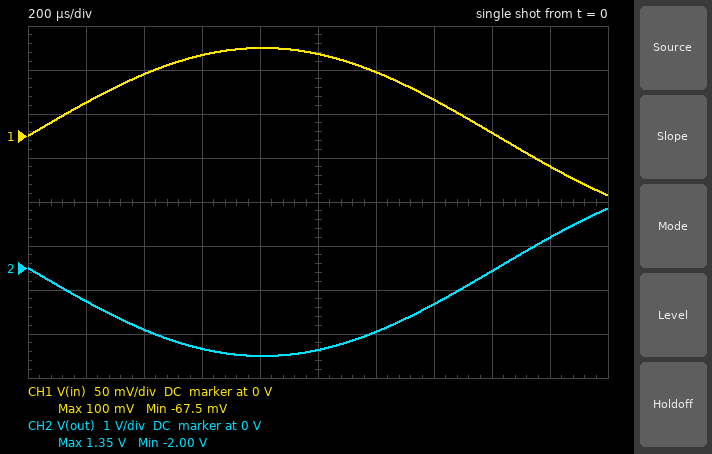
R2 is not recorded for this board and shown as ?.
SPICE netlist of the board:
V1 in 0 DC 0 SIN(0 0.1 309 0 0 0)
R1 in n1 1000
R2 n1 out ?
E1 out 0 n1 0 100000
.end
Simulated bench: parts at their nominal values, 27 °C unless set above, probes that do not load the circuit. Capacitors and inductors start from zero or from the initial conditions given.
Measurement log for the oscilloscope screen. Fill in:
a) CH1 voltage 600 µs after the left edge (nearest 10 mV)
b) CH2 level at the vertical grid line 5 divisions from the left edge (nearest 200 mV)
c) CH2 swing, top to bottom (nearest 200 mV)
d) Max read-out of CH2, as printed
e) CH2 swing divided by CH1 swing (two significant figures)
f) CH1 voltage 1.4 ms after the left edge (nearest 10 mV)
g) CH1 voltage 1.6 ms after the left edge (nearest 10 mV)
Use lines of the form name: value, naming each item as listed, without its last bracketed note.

CH1 voltage 600 µs after the left edge: 90 mV
CH2 level at the vertical grid line 5 divisions from the left edge: -1.8 V
CH2 swing, top to bottom: 3.4 V
Max read-out of CH2, as printed: 1.35 V
CH2 swing divided by CH1 swing: 20
CH1 voltage 1.4 ms after the left edge: 40 mV
CH1 voltage 1.6 ms after the left edge: 0 V
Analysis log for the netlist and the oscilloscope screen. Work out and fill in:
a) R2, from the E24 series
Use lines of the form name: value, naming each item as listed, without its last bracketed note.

R2, from the E24 series: 20 kΩ
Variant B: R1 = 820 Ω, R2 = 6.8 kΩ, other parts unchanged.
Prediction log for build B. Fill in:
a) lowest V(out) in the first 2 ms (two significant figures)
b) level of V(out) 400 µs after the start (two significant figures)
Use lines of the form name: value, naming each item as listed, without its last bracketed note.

lowest V(out) in the first 2 ms: -830 mV
level of V(out) 400 µs after the start: -580 mV
